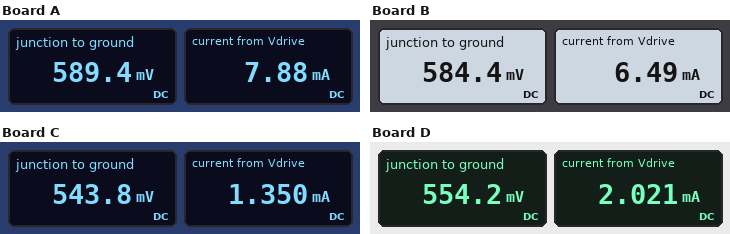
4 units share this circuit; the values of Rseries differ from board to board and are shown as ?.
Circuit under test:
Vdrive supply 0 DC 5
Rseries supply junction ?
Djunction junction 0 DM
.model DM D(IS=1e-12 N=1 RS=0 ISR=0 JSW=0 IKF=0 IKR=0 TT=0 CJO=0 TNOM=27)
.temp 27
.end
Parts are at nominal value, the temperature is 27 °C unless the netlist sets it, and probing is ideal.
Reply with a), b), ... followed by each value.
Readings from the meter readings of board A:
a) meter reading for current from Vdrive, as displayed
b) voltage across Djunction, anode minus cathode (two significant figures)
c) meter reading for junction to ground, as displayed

a) 7.88 mA
b) 590 mV
c) 589.4 mV
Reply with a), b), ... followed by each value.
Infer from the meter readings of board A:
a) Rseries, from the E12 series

a) 560 Ω
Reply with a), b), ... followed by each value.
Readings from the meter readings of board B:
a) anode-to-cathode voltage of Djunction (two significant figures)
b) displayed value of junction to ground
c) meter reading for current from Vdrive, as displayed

a) 580 mV
b) 584.4 mV
c) 6.49 mA
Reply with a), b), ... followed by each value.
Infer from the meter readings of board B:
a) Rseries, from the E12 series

a) 680 Ω
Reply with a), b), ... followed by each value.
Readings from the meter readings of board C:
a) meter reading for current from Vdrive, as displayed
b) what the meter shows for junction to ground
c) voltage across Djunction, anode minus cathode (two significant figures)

a) 1.350 mA
b) 543.8 mV
c) 540 mV
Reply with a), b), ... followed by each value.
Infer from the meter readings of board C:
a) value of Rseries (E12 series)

a) 3.3 kΩ
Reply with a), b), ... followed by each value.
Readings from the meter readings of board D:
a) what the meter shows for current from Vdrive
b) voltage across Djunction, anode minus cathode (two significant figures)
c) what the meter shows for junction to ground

a) 2.021 mA
b) 550 mV
c) 554.2 mV
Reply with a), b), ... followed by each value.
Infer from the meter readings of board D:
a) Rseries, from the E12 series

a) 2.2 kΩ
